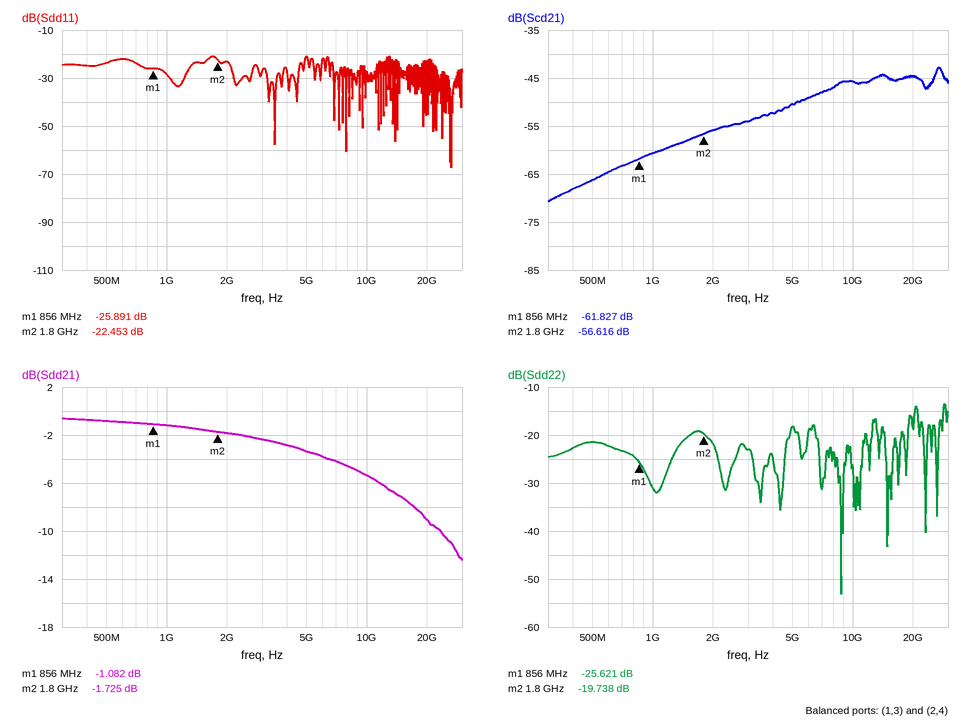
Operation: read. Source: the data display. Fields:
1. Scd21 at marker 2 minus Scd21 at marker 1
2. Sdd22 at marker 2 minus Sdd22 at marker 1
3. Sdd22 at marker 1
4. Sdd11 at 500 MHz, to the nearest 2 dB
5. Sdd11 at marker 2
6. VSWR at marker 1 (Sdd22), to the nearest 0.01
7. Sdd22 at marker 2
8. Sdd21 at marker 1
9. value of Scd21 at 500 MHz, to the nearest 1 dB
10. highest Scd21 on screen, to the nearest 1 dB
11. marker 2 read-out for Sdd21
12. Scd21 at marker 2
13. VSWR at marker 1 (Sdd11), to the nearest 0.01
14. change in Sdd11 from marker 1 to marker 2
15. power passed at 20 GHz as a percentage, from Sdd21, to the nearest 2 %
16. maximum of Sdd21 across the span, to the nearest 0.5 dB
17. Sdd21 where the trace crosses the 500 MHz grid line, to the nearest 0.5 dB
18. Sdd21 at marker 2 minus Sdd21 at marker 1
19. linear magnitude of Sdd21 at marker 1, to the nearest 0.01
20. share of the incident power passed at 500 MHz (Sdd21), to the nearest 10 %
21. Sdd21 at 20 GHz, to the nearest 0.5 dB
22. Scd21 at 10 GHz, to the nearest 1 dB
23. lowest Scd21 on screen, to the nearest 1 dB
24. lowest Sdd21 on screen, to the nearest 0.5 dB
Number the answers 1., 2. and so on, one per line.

1. 5.211 dB
2. 5.883 dB
3. -25.621 dB
4. -24 dB
5. -22.453 dB
6. 1.11
7. -19.738 dB
8. -1.082 dB
9. -66 dB
10. -43 dB
11. -1.725 dB
12. -56.616 dB
13. 1.11
14. 3.438 dB
15. 12 %
16. -0.5 dB
17. -1.0 dB
18. -0.643 dB
19. 0.88
20. 80 %
21. -9.0 dB
22. -46 dB
23. -71 dB
24. -12.5 dB
